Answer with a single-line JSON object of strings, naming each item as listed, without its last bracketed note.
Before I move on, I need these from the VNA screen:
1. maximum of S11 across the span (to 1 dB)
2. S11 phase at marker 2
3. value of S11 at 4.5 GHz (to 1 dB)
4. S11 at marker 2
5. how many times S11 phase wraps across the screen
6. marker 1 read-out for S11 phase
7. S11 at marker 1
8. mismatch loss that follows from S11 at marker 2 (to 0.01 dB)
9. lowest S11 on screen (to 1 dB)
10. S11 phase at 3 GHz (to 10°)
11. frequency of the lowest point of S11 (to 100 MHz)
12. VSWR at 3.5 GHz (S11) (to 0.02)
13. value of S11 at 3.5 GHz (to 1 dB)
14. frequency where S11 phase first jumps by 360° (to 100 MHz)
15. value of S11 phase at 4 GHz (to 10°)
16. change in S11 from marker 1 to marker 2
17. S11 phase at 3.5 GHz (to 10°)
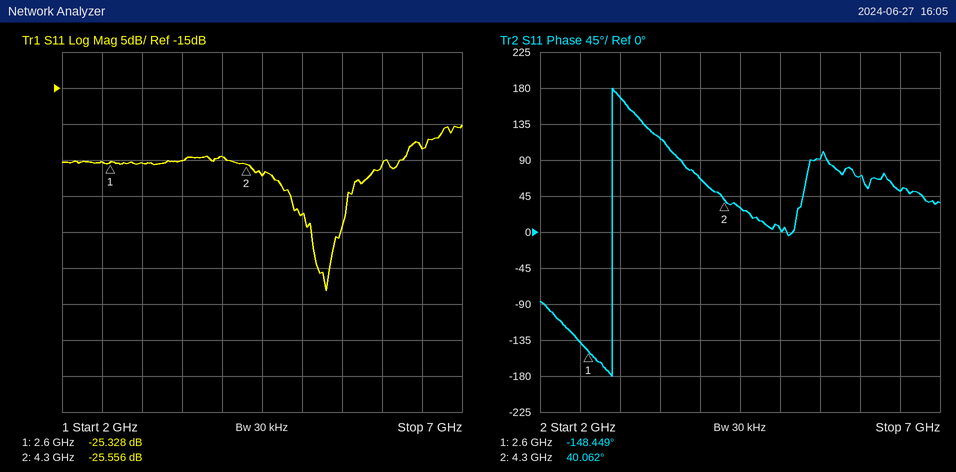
{"maximum of S11 across the span": "-20 dB", "S11 phase at marker 2": "40.062°", "value of S11 at 4.5 GHz": "-27 dB", "S11 at marker 2": "-25.556 dB", "how many times S11 phase wraps across the screen": "1", "marker 1 read-out for S11 phase": "-148.449°", "S11 at marker 1": "-25.328 dB", "mismatch loss that follows from S11 at marker 2": "0.01 dB", "lowest S11 on screen": "-43 dB", "S11 phase at 3 GHz": "170°", "frequency of the lowest point of S11": "5.3 GHz", "VSWR at 3.5 GHz (S11)": "1.12", "value of S11 at 3.5 GHz": "-25 dB", "frequency where S11 phase first jumps by 360°": "2.9 GHz", "value of S11 phase at 4 GHz": "70°", "change in S11 from marker 1 to marker 2": "-0.228 dB", "S11 phase at 3.5 GHz": "120°"}
